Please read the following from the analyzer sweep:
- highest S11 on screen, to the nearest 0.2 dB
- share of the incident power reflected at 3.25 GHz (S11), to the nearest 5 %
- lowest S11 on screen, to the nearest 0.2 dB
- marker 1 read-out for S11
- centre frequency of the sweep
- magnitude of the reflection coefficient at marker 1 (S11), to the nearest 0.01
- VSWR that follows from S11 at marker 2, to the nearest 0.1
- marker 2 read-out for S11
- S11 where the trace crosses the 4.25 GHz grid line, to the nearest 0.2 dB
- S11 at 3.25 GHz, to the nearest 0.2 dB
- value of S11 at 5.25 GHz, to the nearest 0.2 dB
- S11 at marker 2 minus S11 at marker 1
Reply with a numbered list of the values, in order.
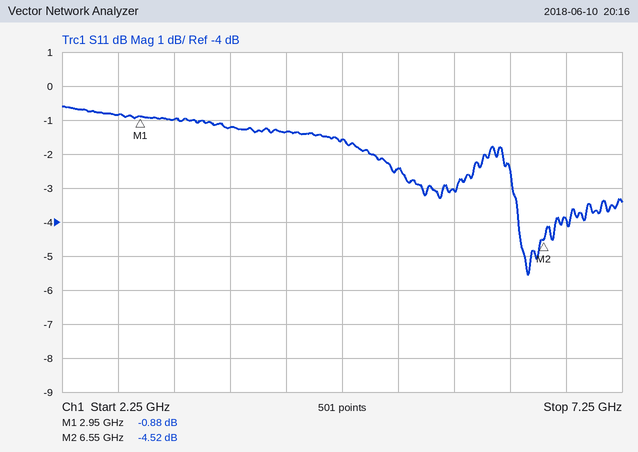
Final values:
1. -0.6 dB
2. 80 %
3. -5.6 dB
4. -0.88 dB
5. 4.75 GHz
6. 0.90
7. 3.9
8. -4.52 dB
9. -1.4 dB
10. -1.0 dB
11. -2.4 dB
12. -3.64 dB
